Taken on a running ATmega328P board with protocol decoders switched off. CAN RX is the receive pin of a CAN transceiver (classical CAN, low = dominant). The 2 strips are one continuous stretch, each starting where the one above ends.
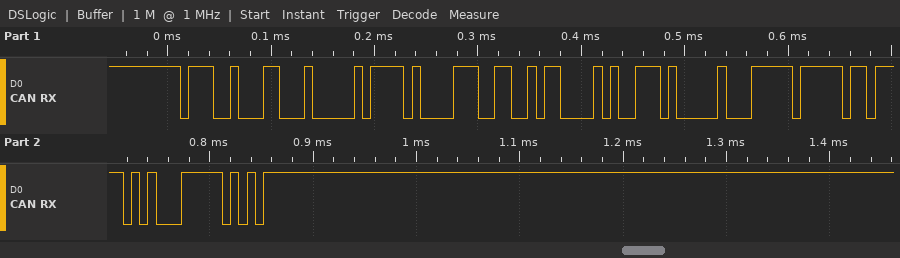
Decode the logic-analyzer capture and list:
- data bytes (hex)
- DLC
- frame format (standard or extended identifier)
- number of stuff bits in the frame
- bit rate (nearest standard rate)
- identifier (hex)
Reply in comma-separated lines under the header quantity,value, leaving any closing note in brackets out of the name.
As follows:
quantity,value
data bytes,1E 87 32 C2 9D 00 FF F7
DLC,8
frame format,standard
number of stuff bits in the frame,5
bit rate,125 kbit/s
identifier,0x723
